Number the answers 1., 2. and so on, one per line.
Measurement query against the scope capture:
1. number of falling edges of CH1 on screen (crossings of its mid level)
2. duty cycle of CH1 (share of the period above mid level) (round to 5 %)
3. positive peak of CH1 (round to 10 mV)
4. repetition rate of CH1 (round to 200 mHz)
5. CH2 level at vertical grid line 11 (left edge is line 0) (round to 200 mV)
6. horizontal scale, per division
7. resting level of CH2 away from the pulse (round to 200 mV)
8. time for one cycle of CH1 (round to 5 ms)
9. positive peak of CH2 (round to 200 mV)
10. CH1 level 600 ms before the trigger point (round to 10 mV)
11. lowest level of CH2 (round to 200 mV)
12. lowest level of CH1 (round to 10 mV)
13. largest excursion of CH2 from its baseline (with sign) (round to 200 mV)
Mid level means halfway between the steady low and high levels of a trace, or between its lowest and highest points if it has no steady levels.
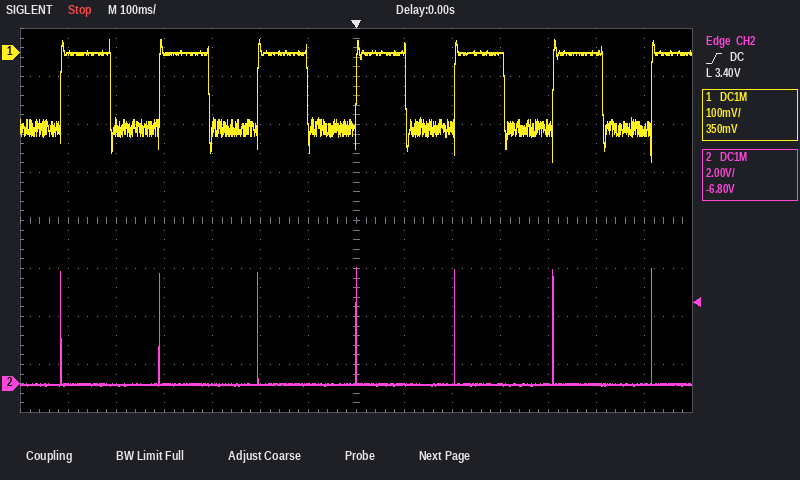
1. 6
2. 50 %
3. 30 mV
4. 4.8 Hz
5. 0.0 V
6. 100 ms
7. 0.0 V
8. 205 ms
9. 4.8 V
10. 0 mV
11. 0.0 V
12. -230 mV
13. +4.8 V
